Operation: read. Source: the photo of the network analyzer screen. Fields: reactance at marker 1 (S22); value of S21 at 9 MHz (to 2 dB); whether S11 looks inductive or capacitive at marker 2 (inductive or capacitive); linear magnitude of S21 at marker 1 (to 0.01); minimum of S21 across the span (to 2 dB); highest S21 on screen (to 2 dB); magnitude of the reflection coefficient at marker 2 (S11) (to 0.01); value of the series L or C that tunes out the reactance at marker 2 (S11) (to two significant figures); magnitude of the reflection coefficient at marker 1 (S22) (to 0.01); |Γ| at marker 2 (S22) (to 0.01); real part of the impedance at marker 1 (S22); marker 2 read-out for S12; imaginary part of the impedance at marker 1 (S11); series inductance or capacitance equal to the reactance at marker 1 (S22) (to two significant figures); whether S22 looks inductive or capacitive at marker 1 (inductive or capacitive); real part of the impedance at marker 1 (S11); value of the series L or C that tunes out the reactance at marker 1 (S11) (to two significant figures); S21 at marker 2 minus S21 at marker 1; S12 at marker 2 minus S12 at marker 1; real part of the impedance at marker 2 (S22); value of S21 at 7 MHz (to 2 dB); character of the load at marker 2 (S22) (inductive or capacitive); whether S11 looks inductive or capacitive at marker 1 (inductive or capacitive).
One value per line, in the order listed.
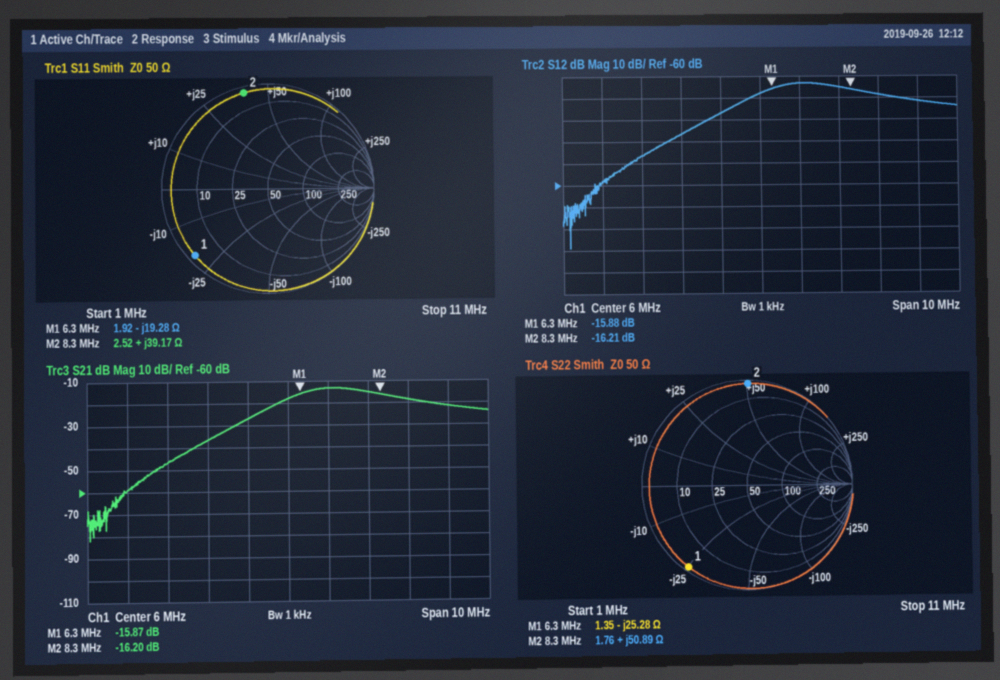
-25.28 Ω
-18 dB
inductive
0.16
-82 dB
-14 dB
0.94
490 pF
0.96
0.97
1.35 Ω
-16.21 dB
-19.28 Ω
1.00 nF
capacitive
1.92 Ω
490 nH
-0.33 dB
-0.33 dB
1.76 Ω
-14 dB
inductive
capacitive
